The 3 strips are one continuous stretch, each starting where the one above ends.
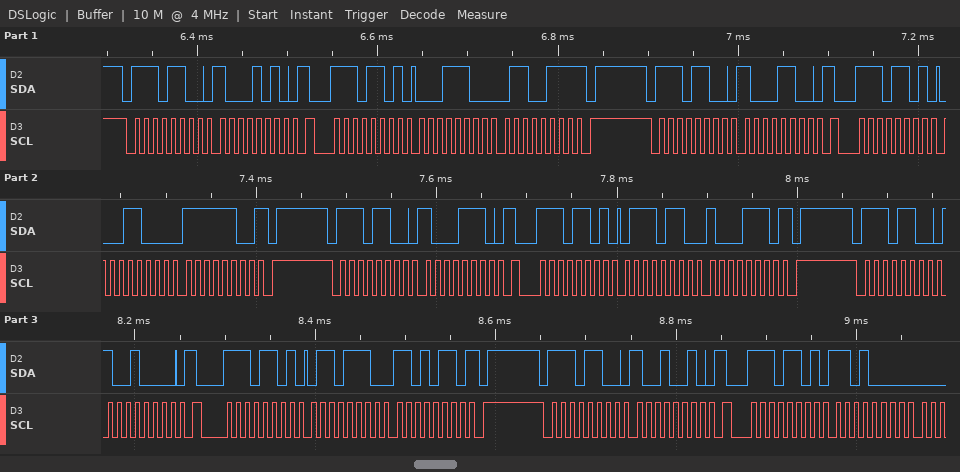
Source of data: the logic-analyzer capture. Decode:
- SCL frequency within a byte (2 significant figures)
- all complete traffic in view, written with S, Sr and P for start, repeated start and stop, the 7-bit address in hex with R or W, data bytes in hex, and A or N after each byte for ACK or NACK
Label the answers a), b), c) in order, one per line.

a) 100 kHz
b) S 76W A 8A A Sr 76R A 1C A 67 N P S 76W A 8C A Sr 76R A 18 A FC N P S 76W A 8E A Sr 76R A 76 A 8E N P S 76W A 90 A Sr 76R A 6E A D6 N P S 76W A 92 A Sr 76R A D0 A
